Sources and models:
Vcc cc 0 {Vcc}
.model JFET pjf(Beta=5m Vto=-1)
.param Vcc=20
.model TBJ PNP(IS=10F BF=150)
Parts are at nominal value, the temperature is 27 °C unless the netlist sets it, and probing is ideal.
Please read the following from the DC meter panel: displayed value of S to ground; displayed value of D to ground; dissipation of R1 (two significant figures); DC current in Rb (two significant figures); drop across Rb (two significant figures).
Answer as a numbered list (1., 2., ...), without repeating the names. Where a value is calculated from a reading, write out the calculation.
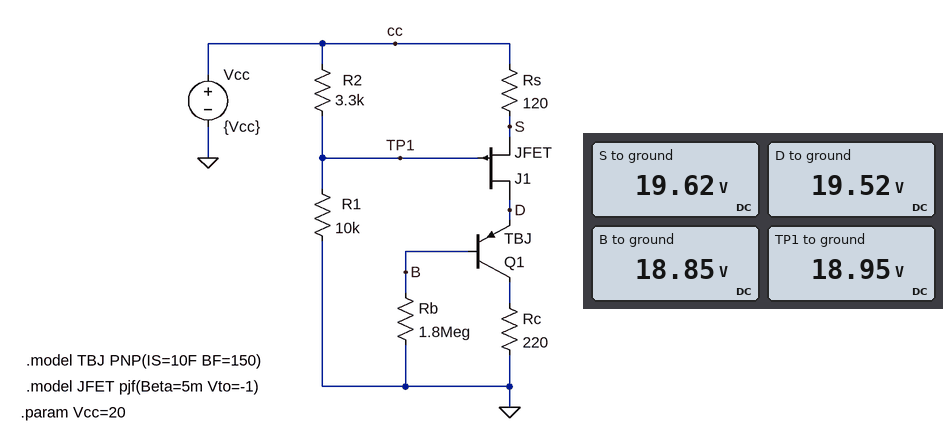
1. 19.62 V
2. 19.52 V
3. (18.95 V)^2 / 10 kΩ = 36 mW
4. (18.85 V) / 1.8 MΩ = 10 µA
5. 18.85 V = 19 V
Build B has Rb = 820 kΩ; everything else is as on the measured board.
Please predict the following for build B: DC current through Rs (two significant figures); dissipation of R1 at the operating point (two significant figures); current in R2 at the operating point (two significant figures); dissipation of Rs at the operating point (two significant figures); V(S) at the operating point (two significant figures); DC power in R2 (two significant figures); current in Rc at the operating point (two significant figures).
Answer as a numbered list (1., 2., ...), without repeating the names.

1. 4.9 mA
2. 35 mW
3. 380 µA
4. 2.9 mW
5. 19 V
6. 480 µW
7. 3.4 mA
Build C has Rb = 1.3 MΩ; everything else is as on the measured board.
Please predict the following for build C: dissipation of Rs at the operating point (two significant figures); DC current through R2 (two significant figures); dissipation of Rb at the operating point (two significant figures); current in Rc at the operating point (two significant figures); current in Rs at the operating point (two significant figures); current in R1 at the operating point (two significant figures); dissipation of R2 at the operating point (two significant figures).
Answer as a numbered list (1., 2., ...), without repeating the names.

1. 1.7 mW
2. 340 µA
3. 270 µW
4. 2.2 mA
5. 3.7 mA
6. 1.9 mA
7. 380 µW
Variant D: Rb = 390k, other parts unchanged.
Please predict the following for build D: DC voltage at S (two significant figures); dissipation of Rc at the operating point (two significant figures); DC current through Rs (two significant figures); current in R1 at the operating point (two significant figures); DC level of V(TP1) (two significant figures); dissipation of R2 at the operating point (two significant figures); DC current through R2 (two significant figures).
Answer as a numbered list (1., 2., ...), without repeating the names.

1. 19 V
2. 10 mW
3. 8.2 mA
4. 1.8 mA
5. 18 V
6. 830 µW
7. 500 µA
